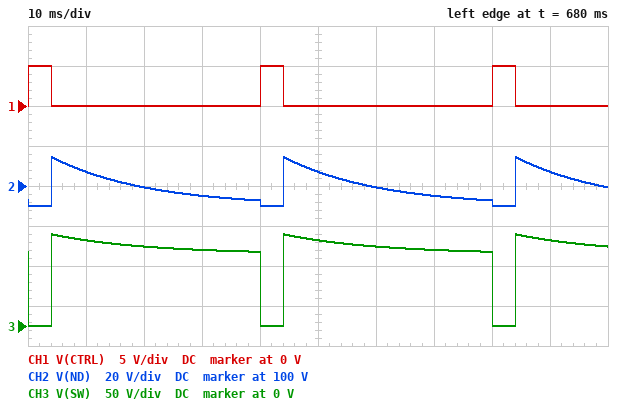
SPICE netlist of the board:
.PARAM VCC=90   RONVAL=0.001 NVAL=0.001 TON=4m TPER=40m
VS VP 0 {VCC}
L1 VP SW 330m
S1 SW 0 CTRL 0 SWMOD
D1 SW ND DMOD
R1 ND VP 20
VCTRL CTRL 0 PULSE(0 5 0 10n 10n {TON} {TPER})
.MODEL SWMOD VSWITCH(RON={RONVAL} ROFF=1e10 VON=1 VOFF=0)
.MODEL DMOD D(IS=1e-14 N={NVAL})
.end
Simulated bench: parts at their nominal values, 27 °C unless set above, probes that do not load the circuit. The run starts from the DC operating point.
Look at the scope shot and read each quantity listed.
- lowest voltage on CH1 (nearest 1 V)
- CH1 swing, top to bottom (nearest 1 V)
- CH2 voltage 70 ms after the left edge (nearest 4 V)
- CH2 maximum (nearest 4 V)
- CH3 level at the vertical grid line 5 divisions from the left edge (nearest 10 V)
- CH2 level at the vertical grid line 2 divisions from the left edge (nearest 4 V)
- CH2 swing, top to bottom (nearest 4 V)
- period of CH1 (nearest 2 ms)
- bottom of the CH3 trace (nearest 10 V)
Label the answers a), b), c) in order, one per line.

a) 0 V
b) 5 V
c) 96 V
d) 116 V
e) 110 V
f) 100 V
g) 24 V
h) 40 ms
i) 0 V
